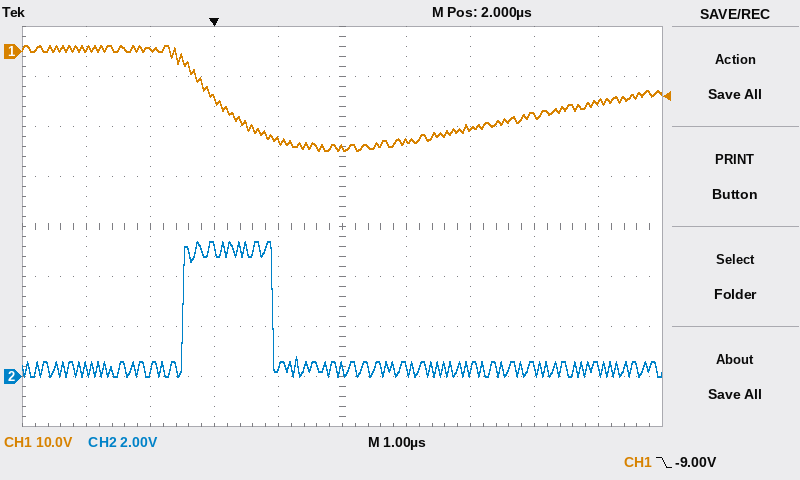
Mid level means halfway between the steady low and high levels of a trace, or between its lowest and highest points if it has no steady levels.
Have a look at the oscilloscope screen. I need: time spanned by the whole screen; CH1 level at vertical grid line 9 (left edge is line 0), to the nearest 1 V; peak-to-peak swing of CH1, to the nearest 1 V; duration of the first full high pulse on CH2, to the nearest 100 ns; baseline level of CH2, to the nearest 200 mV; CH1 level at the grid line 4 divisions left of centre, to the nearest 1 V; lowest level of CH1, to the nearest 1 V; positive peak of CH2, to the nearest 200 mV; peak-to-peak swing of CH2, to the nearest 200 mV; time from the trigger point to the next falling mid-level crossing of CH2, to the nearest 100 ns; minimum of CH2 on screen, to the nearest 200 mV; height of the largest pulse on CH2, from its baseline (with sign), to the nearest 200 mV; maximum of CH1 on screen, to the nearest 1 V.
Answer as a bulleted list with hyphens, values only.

- 10 µs
- -10 V
- 21 V
- 1.4 µs
- 400 mV
- 1 V
- -20 V
- 5.4 V
- 5.4 V
- 900 ns
- 0.0 V
- +5.0 V
- 1 V
